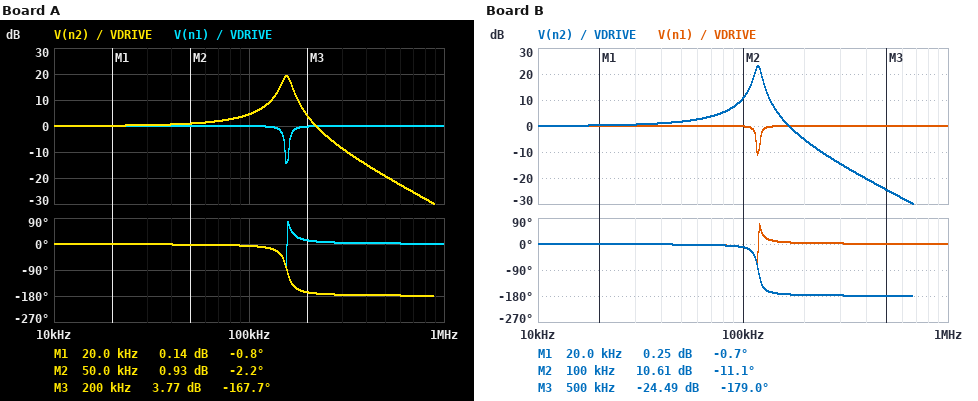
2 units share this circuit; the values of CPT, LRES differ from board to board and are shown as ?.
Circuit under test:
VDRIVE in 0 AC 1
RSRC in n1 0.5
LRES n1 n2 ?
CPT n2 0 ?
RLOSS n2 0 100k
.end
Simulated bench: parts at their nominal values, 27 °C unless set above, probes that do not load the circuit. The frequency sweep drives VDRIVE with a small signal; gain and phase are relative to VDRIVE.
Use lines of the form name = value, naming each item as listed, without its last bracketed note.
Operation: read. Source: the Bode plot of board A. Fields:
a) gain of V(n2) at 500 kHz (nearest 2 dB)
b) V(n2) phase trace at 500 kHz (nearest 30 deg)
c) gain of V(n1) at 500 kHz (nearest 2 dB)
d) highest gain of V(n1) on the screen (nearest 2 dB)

gain of V(n2) at 500 kHz = -20 dB
V(n2) phase trace at 500 kHz = -180 deg
gain of V(n1) at 500 kHz = 0 dB
highest gain of V(n1) on the screen = 0 dB
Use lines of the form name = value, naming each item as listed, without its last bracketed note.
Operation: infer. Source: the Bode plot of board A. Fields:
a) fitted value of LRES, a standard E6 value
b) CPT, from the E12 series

fitted value of LRES, a standard E6 value = 4.7 µH
CPT, from the E12 series = 220 nF
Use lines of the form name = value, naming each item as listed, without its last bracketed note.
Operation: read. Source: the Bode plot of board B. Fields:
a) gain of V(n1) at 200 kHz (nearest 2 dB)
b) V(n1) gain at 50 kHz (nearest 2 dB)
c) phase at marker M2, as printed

gain of V(n1) at 200 kHz = 0 dB
V(n1) gain at 50 kHz = 0 dB
phase at marker M2, as printed = -11.1 deg
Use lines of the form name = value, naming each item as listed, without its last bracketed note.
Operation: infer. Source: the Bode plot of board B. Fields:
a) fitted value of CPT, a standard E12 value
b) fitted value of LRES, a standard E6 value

fitted value of CPT, a standard E12 value = 180 nF
fitted value of LRES, a standard E6 value = 10 µH
